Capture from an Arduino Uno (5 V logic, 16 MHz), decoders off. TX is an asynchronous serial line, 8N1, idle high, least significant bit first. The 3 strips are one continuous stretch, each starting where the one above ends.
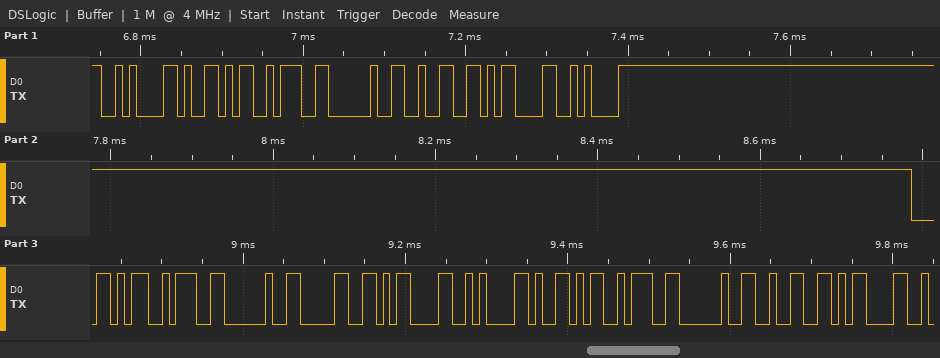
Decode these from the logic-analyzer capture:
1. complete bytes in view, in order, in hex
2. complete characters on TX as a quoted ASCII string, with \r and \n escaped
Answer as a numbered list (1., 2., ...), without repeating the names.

1. 0A 59 3A 20 32 0D 0A 58 3A 20 30 0D 0A 59 3A 20 32 0D
2. "\nY: 2\r\nX: 0\r\nY: 2\r"
